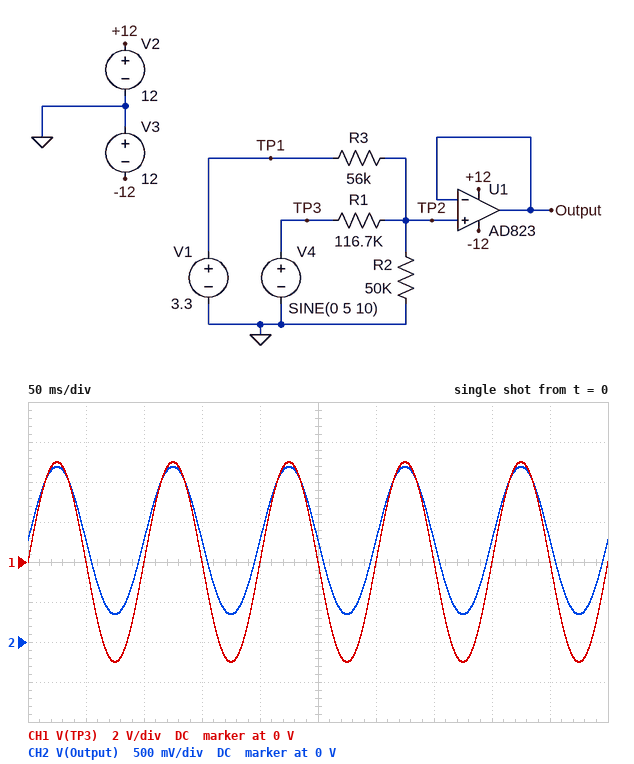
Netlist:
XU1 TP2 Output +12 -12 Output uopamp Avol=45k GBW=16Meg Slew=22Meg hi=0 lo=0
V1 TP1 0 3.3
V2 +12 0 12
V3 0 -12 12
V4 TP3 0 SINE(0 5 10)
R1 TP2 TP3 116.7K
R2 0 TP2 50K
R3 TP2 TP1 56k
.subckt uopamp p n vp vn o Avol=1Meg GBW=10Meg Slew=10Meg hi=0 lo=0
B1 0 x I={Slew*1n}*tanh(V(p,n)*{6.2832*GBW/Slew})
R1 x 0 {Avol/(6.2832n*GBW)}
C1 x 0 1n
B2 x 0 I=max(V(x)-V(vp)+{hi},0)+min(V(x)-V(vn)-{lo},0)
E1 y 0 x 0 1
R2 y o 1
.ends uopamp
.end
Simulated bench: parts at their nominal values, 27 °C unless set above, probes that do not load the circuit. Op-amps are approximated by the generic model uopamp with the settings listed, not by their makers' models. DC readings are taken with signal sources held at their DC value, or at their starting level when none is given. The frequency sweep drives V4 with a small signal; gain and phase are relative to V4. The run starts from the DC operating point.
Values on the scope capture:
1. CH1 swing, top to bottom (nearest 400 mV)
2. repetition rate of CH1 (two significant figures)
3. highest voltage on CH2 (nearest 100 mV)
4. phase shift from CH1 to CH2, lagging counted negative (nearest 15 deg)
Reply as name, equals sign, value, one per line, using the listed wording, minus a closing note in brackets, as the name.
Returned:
CH1 swing, top to bottom = 10.0 V
repetition rate of CH1 = 10 Hz
highest voltage on CH2 = 2.2 V
phase shift from CH1 to CH2, lagging counted negative = 0 deg
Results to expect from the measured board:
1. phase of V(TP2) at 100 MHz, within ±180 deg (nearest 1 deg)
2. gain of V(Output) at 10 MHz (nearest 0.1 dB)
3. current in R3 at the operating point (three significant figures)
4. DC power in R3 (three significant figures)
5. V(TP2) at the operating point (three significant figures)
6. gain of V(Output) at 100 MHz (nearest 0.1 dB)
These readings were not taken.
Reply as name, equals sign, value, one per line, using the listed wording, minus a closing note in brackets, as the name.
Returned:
phase of V(TP2) at 100 MHz, within ±180 deg = 0 deg
gain of V(Output) at 10 MHz = -16.1 dB
current in R3 at the operating point = 36.3 µA
DC power in R3 = 73.6 µW
V(TP2) at the operating point = 1.27 V
gain of V(Output) at 100 MHz = -30.7 dB
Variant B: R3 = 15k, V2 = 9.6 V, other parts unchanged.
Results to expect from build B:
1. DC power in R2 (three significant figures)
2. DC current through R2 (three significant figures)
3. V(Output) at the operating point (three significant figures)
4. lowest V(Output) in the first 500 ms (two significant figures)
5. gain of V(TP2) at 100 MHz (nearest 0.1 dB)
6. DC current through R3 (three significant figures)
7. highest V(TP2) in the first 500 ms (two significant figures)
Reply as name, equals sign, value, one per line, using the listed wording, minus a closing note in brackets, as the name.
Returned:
DC power in R2 = 107 µW
DC current through R2 = 46.2 µA
V(Output) at the operating point = 2.31 V
lowest V(Output) in the first 500 ms = 1.9 V
gain of V(TP2) at 100 MHz = -20.9 dB
DC current through R3 = 66.0 µA
highest V(TP2) in the first 500 ms = 2.8 V
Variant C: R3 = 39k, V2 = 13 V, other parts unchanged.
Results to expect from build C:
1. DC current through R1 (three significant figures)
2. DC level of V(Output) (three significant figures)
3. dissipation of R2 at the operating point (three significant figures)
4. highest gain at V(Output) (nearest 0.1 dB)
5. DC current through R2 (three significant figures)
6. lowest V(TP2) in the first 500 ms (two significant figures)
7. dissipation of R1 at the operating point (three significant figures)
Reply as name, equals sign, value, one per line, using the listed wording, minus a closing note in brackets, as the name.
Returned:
DC current through R1 = 13.4 µA
DC level of V(Output) = 1.56 V
dissipation of R2 at the operating point = 48.7 µW
highest gain at V(Output) = -16.0 dB
DC current through R2 = 31.2 µA
lowest V(TP2) in the first 500 ms = 770 mV
dissipation of R1 at the operating point = 20.9 µW
